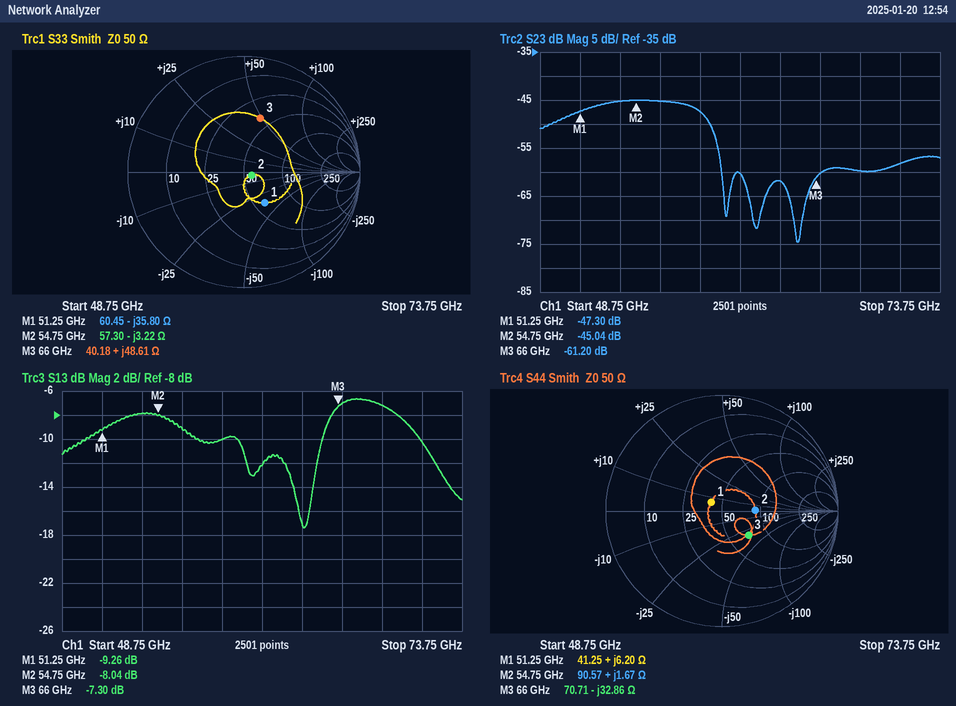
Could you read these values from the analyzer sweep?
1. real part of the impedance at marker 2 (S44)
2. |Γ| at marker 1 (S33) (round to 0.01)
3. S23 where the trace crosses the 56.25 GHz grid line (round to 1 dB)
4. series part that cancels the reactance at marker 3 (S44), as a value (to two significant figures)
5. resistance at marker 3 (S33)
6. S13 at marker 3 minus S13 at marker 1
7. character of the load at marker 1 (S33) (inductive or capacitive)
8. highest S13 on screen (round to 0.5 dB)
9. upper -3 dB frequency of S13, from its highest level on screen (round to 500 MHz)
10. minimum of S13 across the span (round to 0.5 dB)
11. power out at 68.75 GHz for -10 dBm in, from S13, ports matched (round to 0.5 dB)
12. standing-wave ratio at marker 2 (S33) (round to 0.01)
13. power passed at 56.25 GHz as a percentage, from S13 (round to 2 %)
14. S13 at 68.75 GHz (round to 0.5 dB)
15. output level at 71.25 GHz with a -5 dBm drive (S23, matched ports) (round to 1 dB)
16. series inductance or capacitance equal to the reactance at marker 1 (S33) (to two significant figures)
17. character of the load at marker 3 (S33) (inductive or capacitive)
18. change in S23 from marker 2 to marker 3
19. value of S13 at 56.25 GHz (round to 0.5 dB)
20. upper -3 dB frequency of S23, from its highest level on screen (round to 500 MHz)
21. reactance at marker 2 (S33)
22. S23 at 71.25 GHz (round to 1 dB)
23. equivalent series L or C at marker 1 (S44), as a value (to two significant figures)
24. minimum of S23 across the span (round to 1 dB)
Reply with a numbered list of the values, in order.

1. 90.57 Ω
2. 0.32
3. -45 dB
4. 79 pH
5. 40.18 Ω
6. 1.96 dB
7. capacitive
8. -6.5 dB
9. 71.0 GHz
10. -17.5 dB
11. -17.0 dBm
12. 1.16
13. 12 %
14. -7.0 dB
15. -63 dBm
16. 87 fF
17. inductive
18. -16.16 dB
19. -9.0 dB
20. 59.0 GHz
21. -3.22 Ω
22. -58 dB
23. 19 pH
24. -75 dB
